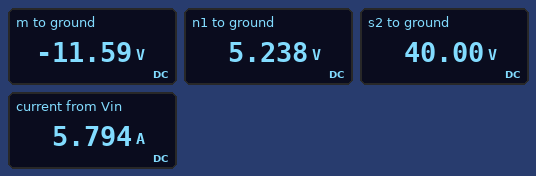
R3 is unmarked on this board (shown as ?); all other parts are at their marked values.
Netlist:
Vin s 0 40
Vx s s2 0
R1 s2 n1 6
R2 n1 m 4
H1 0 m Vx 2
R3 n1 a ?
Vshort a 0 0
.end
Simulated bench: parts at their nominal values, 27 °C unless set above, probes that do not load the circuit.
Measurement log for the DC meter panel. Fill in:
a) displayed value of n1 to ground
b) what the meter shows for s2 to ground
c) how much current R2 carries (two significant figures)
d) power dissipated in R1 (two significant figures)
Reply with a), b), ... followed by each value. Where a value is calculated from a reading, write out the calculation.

a) 5.238 V
b) 40.00 V
c) (5.238 V - (-11.59 V)) / 4 Ω = 4.2 A
d) (40 V - 5.238 V)^2 / 6 Ω = 200 W
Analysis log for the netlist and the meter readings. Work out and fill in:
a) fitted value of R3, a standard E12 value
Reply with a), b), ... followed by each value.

a) 3.3 Ω
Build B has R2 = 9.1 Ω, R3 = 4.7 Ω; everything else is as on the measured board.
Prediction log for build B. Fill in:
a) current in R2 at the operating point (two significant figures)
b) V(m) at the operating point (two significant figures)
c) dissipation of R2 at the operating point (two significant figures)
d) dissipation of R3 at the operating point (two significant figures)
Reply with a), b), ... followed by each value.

a) 2.3 A
b) -9.5 V
c) 48 W
d) 28 W
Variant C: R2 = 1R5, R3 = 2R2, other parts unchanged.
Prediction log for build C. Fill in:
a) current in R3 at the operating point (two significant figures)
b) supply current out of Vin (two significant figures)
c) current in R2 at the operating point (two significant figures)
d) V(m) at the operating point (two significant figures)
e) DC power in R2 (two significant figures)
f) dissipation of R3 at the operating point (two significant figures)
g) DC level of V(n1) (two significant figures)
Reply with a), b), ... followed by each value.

a) 950 mA
b) 7.0 A
c) 8.0 A
d) -14 V
e) 95 W
f) 2.0 W
g) -2.1 V
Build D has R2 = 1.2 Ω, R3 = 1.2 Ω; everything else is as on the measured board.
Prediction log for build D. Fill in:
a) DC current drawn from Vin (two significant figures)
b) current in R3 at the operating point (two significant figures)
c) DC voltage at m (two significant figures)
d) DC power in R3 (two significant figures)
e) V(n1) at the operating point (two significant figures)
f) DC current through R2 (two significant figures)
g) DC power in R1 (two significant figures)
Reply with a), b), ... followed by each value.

a) 7.1 A
b) 2.4 A
c) -14 V
d) 6.8 W
e) -2.9 V
f) 9.5 A
g) 310 W
